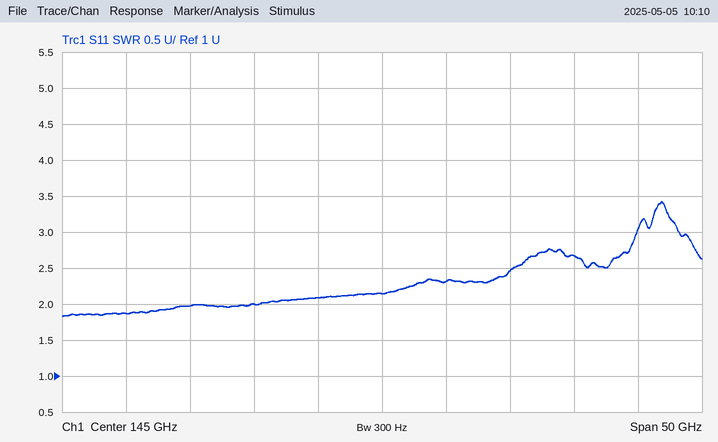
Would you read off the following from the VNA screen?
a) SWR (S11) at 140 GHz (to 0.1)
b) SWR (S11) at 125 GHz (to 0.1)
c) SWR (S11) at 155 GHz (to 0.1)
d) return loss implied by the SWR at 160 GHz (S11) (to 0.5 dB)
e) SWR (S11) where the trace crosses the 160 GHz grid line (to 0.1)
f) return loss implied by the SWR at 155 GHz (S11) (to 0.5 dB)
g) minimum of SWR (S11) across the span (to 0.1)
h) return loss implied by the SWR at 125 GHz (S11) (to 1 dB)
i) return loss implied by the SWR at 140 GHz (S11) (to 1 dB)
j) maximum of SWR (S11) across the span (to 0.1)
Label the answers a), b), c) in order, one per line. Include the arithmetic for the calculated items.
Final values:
a) 2.1
b) 1.9
c) 2.5
d) −20 log10((2.7 − 1)/(2.7 + 1)) ≈ 6.76 dB, so 7.0 dB to the nearest 0.5 dB
e) 2.7
f) −20 log10((2.5 − 1)/(2.5 + 1)) ≈ 7.36 dB, so 7.5 dB to the nearest 0.5 dB
g) 1.8
h) −20 log10((1.9 − 1)/(1.9 + 1)) ≈ 10 dB
i) −20 log10((2.1 − 1)/(2.1 + 1)) ≈ 9 dB
j) 3.4
